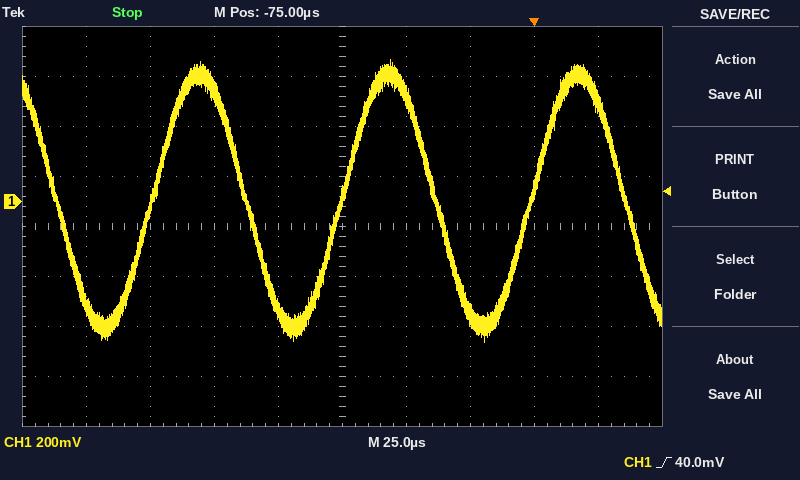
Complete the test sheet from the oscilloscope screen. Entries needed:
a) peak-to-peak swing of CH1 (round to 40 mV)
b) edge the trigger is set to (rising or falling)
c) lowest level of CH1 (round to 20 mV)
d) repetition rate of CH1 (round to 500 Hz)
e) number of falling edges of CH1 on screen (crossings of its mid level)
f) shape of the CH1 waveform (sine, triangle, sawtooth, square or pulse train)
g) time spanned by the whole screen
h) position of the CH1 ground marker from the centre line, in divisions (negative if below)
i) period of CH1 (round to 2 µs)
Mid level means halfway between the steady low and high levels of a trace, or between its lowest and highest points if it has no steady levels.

1.12 V
rising
-560 mV
13.5 kHz
4
sine
250 µs
+0.5 div
74 µs
